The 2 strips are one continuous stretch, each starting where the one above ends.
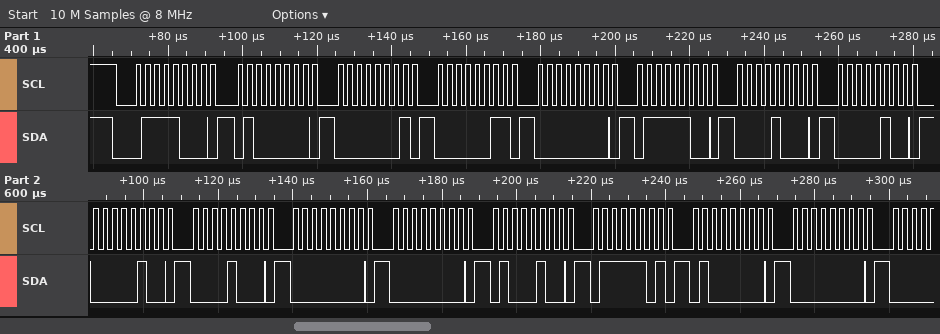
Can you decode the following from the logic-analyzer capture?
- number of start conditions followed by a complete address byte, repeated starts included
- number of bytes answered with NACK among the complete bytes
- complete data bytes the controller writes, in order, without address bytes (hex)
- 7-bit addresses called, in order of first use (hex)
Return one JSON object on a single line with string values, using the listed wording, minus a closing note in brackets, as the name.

{"number of start conditions followed by a complete address byte, repeated starts included": "1", "number of bytes answered with NACK among the complete bytes": "0", "complete data bytes the controller writes, in order, without address bytes": "40 01 03 00 7C 08 04 04 08 00 00 44 7D 40 00", "7-bit addresses called, in order of first use": "0x3C"}
